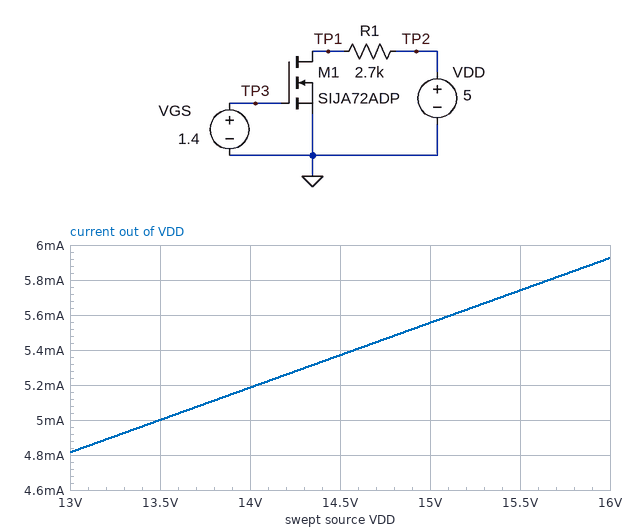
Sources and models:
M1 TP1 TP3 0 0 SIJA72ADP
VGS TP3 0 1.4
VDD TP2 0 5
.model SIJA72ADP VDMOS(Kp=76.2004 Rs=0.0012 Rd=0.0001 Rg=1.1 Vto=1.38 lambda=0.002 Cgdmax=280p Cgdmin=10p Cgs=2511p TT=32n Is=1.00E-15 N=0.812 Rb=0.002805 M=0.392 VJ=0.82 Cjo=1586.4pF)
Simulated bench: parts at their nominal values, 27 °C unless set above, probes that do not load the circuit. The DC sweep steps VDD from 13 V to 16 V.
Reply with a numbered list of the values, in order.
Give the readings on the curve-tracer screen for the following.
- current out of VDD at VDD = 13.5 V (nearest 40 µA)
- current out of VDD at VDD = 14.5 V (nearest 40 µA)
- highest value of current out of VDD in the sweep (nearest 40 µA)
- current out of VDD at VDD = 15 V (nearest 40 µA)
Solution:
1. 5.00 mA
2. 5.36 mA
3. 5.92 mA
4. 5.56 mA
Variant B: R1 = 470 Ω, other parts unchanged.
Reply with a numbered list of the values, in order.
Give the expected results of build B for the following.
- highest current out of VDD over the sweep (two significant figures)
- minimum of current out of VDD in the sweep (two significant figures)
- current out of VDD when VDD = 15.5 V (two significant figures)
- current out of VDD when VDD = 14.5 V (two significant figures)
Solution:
1. 34 mA
2. 28 mA
3. 33 mA
4. 31 mA
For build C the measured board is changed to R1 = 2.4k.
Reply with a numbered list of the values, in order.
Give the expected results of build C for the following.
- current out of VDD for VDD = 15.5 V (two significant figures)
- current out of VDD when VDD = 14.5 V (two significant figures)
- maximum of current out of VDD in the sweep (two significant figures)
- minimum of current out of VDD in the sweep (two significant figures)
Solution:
1. 6.5 mA
2. 6.0 mA
3. 6.7 mA
4. 5.4 mA
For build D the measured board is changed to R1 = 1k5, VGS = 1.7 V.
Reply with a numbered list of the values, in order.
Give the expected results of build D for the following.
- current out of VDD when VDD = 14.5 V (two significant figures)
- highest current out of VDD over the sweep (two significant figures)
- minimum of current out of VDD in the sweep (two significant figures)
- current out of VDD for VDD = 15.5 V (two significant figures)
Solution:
1. 9.7 mA
2. 11 mA
3. 8.7 mA
4. 10 mA
